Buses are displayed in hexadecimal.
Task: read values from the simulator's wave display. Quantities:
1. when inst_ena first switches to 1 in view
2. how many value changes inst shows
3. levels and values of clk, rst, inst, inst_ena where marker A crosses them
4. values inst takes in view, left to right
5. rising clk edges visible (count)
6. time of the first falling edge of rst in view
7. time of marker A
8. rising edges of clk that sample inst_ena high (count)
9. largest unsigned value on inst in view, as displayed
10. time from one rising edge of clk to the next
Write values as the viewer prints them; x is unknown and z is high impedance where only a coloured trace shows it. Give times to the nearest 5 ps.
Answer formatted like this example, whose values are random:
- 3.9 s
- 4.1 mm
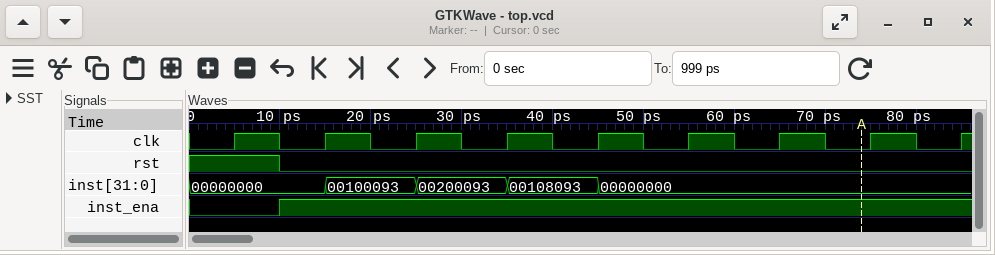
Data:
- 10 ps
- 4
- clk=0, rst=0, inst=00000000, inst_ena=1
- 00000000, 00100093, 00200093, 00108093, 00000000
- 9
- 10 ps
- 75 ps
- 8
- 00200093
- 10 ps
